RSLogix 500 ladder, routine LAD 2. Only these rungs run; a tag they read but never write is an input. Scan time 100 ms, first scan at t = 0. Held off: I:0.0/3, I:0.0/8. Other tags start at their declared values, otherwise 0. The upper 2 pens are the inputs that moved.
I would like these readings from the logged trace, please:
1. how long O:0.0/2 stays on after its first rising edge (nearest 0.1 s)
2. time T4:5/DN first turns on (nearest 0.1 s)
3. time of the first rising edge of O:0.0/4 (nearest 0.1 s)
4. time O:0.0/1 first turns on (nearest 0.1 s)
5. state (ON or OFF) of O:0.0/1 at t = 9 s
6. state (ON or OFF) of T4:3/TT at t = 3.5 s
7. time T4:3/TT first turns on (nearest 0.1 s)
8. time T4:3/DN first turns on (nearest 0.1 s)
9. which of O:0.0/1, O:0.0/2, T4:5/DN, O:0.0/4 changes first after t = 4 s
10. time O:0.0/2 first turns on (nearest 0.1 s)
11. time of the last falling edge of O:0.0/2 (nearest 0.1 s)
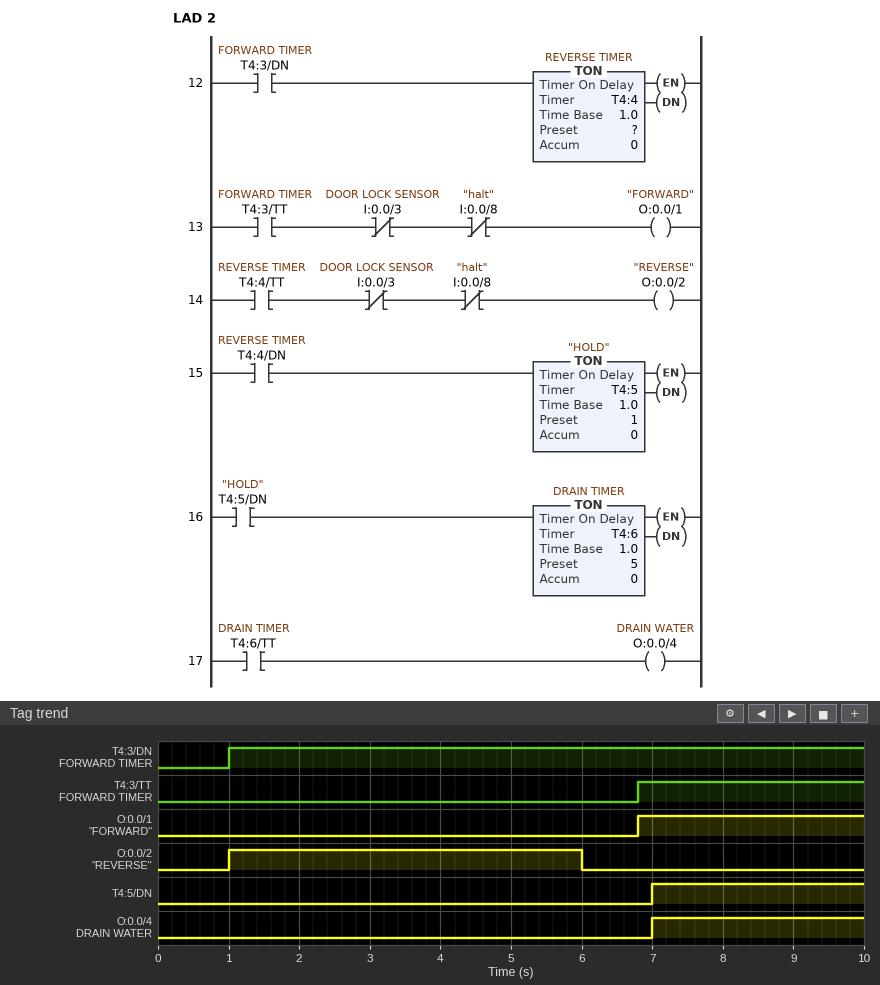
5.0 s
7.0 s
7.0 s
6.8 s
ON
OFF
6.8 s
1.0 s
O:0.0/2
1.0 s
6.0 s
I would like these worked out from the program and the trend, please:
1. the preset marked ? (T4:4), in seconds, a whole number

5 s
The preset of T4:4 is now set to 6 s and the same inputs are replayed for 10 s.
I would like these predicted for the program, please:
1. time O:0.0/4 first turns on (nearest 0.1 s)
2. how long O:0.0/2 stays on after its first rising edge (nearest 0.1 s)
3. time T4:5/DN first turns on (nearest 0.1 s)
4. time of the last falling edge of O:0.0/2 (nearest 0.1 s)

8.0 s
6.0 s
8.0 s
7.0 s
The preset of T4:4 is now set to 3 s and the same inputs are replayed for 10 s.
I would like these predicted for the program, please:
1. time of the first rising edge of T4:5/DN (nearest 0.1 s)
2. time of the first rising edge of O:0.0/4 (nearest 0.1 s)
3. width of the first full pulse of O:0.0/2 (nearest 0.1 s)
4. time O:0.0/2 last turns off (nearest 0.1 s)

5.0 s
5.0 s
3.0 s
4.0 s
